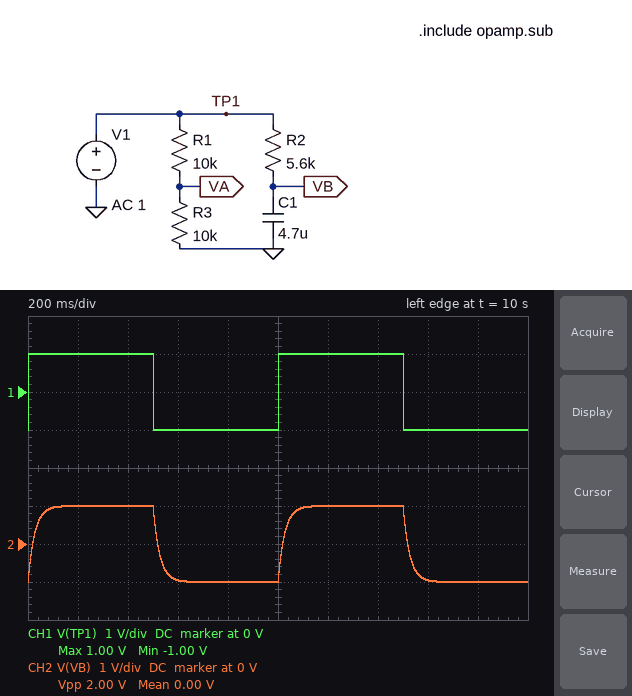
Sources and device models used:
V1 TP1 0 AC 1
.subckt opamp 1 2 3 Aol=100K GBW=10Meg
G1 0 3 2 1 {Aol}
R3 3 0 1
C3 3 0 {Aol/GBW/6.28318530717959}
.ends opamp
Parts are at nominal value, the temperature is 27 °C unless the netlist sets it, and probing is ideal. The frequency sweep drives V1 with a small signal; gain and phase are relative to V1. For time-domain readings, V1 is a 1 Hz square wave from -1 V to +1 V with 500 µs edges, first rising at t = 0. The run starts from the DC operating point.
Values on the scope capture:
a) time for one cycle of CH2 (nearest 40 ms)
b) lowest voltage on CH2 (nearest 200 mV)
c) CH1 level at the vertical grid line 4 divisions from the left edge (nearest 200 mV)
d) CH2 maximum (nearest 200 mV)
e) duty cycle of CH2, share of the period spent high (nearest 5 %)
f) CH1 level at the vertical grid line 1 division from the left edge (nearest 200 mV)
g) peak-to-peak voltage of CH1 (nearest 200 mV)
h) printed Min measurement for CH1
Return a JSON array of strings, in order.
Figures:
["1.00 s", "-1.0 V", "-1.0 V", "1.0 V", "50 %", "1.0 V", "2.0 V", "-1.00 V"]
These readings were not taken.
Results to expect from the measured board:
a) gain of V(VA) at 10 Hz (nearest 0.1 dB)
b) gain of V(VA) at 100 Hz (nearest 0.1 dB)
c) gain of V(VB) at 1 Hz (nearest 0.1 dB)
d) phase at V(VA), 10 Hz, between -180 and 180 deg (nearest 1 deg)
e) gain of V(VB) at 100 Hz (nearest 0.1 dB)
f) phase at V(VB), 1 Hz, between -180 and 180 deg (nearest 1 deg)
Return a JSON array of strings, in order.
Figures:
["-6.0 dB", "-6.0 dB", "-0.1 dB", "0 deg", "-24.4 dB", "-9 deg"]
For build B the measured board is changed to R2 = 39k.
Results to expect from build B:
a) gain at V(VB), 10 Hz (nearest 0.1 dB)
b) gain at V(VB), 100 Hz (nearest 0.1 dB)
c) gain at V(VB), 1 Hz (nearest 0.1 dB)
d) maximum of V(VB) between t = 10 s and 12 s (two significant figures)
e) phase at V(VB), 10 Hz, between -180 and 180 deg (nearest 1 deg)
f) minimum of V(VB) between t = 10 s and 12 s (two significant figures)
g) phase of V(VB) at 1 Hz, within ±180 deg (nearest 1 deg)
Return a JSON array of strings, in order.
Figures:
["-21.3 dB", "-41.2 dB", "-3.7 dB", "880 mV", "-85 deg", "-880 mV", "-49 deg"]
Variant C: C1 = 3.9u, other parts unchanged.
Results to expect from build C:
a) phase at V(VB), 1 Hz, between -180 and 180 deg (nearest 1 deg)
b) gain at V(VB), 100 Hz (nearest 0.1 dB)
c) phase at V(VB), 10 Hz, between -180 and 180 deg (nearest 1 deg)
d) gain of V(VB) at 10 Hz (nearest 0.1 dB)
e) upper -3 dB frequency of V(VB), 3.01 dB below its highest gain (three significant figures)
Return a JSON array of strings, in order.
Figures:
["-8 deg", "-22.8 dB", "-54 deg", "-4.6 dB", "7.29 Hz"]
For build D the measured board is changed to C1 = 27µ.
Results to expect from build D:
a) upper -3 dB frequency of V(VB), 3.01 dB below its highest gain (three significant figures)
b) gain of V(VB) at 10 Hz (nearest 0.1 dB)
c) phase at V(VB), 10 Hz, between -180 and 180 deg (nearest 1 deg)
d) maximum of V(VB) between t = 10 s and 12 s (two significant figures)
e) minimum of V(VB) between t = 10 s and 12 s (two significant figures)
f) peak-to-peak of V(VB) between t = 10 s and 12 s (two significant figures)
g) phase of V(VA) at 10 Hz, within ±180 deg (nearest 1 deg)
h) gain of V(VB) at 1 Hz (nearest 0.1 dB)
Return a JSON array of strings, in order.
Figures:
["1.05 Hz", "-19.6 dB", "-84 deg", "930 mV", "-930 mV", "1.9 V", "0 deg", "-2.8 dB"]
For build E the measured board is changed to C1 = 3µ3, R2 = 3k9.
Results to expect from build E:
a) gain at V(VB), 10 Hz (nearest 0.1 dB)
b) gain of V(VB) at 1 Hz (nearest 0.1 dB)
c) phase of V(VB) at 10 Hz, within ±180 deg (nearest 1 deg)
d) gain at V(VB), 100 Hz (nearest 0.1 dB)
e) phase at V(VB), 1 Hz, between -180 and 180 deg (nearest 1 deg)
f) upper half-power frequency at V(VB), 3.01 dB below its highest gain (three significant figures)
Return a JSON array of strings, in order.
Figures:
["-2.2 dB", "0 dB", "-39 deg", "-18.2 dB", "-5 deg", "12.4 Hz"]
